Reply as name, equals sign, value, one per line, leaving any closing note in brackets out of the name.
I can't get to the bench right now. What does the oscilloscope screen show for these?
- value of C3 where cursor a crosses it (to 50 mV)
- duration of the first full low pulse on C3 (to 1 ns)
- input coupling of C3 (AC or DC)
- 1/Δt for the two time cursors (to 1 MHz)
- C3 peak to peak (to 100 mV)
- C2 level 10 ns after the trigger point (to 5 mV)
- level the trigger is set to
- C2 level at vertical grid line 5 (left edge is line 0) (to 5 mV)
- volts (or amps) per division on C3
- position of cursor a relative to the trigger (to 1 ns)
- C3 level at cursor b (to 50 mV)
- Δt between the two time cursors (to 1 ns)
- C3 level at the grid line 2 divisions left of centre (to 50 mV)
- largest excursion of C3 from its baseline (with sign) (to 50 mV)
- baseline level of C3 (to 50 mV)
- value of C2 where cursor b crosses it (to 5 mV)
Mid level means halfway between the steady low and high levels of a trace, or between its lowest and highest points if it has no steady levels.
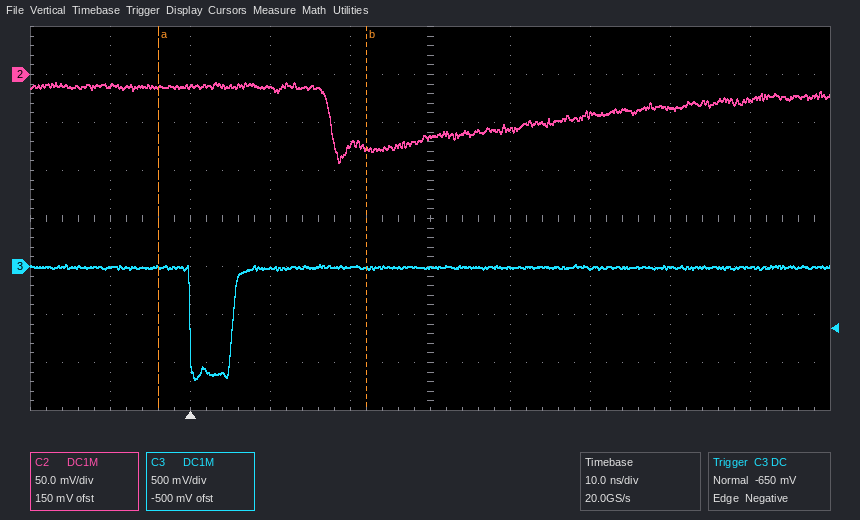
value of C3 where cursor a crosses it = 0 mV
duration of the first full low pulse on C3 = 5 ns
input coupling of C3 = DC
1/Δt for the two time cursors = 38 MHz
C3 peak to peak = 1.20 V
C2 level 10 ns after the trigger point = -15 mV
level the trigger is set to = -650 mV
C2 level at vertical grid line 5 (left edge is line 0) = -65 mV
volts (or amps) per division on C3 = 500 mV
position of cursor a relative to the trigger = -4 ns
C3 level at cursor b = 0 mV
Δt between the two time cursors = 26 ns
C3 level at the grid line 2 divisions left of centre = 0 mV
largest excursion of C3 from its baseline (with sign) = -1.15 V
baseline level of C3 = 0 mV
value of C2 where cursor b crosses it = -75 mV
